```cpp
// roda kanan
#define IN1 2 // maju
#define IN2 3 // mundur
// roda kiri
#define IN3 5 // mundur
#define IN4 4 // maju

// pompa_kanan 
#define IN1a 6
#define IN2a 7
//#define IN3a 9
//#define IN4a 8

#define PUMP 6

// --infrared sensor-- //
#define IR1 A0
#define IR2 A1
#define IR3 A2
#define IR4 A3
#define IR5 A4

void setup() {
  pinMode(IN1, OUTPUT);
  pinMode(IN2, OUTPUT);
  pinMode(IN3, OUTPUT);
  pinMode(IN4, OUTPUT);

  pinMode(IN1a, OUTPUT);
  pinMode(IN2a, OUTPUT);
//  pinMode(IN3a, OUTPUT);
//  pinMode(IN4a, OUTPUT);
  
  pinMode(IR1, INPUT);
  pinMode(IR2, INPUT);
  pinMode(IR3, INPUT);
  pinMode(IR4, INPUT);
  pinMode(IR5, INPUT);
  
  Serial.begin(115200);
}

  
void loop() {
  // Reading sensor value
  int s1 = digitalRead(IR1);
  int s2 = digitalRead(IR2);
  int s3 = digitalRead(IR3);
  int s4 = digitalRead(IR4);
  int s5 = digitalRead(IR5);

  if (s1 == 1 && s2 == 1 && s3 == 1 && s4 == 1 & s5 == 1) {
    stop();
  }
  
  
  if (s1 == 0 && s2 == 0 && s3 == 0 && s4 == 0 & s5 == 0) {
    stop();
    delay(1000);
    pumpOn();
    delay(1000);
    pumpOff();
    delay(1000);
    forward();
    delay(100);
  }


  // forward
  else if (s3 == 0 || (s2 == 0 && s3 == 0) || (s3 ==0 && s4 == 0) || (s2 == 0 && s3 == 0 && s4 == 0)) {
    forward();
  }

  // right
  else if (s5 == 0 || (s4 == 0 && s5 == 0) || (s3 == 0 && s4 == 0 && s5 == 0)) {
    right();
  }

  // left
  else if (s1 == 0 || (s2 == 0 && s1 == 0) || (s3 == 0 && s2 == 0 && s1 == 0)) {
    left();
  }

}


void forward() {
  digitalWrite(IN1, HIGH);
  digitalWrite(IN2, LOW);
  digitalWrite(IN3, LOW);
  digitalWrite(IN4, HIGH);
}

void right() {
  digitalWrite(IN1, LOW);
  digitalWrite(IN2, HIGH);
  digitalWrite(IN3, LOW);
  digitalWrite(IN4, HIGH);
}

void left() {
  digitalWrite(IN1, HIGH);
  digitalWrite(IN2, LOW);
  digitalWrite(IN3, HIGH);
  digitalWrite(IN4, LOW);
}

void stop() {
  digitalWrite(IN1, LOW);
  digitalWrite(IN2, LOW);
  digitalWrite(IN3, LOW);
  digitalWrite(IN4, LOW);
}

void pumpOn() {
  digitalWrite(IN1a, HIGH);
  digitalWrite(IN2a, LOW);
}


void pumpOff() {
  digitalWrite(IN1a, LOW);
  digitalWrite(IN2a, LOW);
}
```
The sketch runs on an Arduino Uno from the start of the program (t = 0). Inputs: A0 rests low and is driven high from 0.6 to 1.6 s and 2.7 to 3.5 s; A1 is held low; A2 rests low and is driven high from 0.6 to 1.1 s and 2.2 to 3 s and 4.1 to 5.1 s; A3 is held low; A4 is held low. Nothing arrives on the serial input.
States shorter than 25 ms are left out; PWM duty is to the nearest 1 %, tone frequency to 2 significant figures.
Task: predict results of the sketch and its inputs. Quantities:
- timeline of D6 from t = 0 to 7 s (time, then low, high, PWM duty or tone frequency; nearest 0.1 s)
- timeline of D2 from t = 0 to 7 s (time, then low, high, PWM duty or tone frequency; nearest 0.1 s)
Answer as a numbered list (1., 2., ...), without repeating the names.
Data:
1. 0 s low; 1 s high; 2 s low; 4.5 s high; 5.5 s low
2. 0 s low; 3 s high; 3.5 s low; 6.5 s high; 6.6 s low
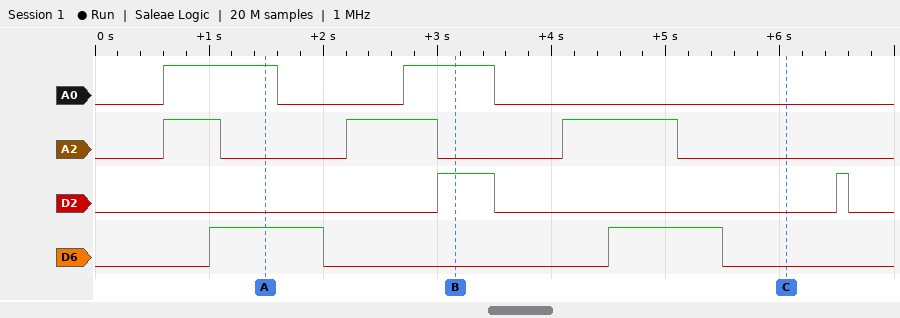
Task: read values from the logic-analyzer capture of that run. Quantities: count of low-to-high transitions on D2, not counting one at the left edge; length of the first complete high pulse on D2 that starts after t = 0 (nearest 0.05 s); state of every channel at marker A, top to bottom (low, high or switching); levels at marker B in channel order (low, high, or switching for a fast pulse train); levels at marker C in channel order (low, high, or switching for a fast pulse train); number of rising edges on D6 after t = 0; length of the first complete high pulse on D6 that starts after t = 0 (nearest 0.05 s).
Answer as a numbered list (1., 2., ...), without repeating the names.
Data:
1. 2
2. 0.50 s
3. A0 high, A2 low, D2 low, D6 high
4. A0 high, A2 low, D2 high, D6 low
5. A0 low, A2 low, D2 low, D6 low
6. 2
7. 1.00 s
